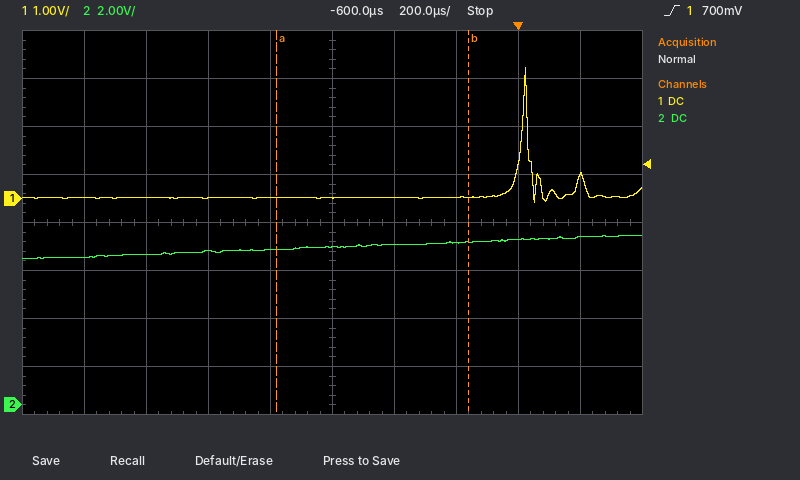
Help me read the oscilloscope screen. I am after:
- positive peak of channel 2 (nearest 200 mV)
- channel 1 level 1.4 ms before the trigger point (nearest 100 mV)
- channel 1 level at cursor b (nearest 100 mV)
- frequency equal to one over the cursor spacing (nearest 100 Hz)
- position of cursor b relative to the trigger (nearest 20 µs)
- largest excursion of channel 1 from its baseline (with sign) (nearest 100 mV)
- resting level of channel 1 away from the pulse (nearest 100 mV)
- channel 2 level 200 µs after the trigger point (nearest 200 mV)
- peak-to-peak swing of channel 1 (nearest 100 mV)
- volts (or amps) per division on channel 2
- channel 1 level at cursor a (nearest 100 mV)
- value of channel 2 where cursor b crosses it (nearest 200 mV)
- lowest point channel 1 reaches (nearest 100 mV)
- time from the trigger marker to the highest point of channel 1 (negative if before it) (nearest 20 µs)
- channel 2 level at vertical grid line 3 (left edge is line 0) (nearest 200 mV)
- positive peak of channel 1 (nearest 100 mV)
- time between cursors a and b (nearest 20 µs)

7.0 V
0.0 V
0.0 V
1.6 kHz
-160 µs
+2.7 V
0.0 V
7.0 V
2.8 V
2 V
0.0 V
6.8 V
-100 mV
+20 µs
6.4 V
2.7 V
620 µs
